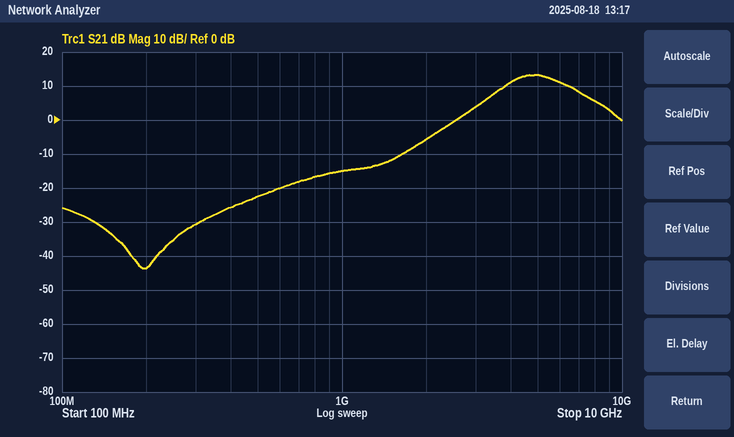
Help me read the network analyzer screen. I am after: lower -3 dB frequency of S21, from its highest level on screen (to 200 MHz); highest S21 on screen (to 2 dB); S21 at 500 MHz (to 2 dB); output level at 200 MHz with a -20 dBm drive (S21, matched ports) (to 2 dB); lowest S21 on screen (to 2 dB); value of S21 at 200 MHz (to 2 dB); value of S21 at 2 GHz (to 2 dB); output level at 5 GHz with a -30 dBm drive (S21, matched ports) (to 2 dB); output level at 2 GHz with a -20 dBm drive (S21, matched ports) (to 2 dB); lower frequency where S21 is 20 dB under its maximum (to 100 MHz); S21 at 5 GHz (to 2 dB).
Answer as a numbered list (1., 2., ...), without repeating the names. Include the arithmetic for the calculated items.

1. 3.8 GHz
2. 14 dB
3. -22 dB
4. -20 dBm + (-44 dB) = -64 dBm
5. -44 dB
6. -44 dB
7. -6 dB
8. -30 dBm + (14 dB) = -16 dBm
9. -20 dBm + (-6 dB) = -26 dBm
10. 1.9 GHz
11. 14 dB
